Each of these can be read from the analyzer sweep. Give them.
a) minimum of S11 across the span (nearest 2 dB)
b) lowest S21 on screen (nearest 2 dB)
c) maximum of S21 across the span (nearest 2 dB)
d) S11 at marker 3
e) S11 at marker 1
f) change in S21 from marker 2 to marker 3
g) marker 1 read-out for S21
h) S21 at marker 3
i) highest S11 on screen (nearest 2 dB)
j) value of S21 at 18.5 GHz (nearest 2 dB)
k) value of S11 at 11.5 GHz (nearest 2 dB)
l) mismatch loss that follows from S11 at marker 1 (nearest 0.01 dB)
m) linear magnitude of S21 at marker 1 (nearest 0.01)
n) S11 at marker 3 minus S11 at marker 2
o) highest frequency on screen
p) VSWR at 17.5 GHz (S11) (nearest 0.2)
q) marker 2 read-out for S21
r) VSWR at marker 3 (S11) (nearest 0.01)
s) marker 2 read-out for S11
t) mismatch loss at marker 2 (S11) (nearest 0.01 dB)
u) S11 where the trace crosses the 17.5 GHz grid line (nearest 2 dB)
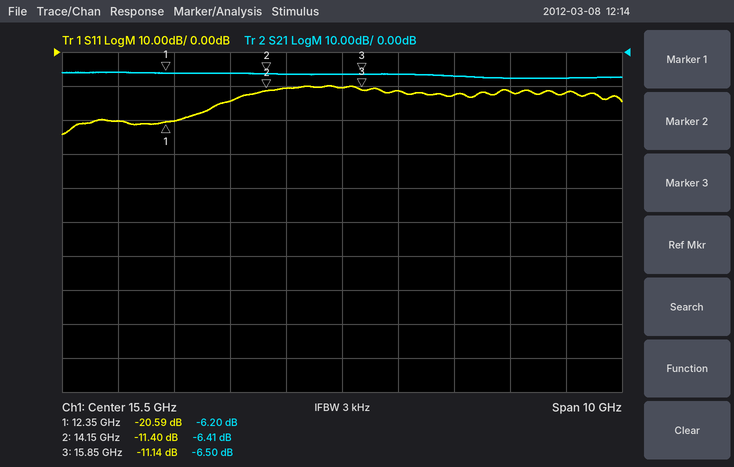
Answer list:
-24 dB
-8 dB
-6 dB
-11.14 dB
-20.59 dB
-0.09 dB
-6.20 dB
-6.50 dB
-10 dB
-8 dB
-20 dB
0.04 dB
0.49
0.26 dB
20.5 GHz
1.6
-6.41 dB
1.77
-11.40 dB
0.33 dB
-12 dB
